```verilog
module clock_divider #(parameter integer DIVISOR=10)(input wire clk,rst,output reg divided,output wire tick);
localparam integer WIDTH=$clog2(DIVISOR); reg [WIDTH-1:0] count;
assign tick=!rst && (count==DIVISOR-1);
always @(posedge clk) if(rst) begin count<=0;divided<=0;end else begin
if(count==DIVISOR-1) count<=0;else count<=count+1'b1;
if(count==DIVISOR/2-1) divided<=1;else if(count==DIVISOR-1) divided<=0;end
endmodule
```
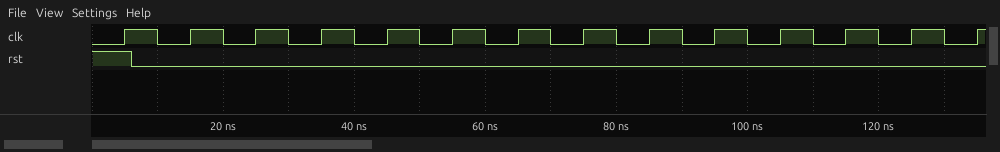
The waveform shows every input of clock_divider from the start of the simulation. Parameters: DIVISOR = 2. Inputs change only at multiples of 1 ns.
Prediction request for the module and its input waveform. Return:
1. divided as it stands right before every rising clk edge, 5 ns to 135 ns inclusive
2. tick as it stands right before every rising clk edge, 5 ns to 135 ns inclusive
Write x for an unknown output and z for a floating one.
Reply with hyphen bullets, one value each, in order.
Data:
- x 0 1 0 1 0 1 0 1 0 1 0 1 0
- 0 0 1 0 1 0 1 0 1 0 1 0 1 0
